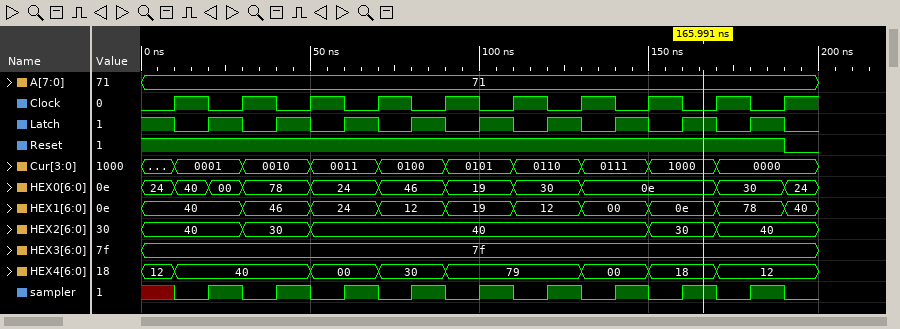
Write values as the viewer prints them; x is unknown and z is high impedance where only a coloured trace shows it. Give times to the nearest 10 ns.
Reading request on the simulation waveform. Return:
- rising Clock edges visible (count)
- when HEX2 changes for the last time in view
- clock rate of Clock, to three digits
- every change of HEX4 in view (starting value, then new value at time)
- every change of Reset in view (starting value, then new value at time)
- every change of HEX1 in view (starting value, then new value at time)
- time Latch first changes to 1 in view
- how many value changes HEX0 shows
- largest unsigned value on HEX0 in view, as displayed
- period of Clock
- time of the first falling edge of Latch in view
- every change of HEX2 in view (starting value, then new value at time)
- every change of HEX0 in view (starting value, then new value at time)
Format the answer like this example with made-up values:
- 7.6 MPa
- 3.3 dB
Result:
- 10
- 170 ns
- 50.0 MHz
- 12, 40 at 10 ns, 00 at 50 ns, 30 at 70 ns, 79 at 90 ns, 00 at 130 ns, 18 at 150 ns, 12 at 170 ns
- 1, 0 at 190 ns
- 40, 46 at 30 ns, 24 at 50 ns, 12 at 70 ns, 19 at 90 ns, 12 at 110 ns, 00 at 130 ns, 0e at 150 ns, 78 at 170 ns, 40 at 190 ns
- 20 ns
- 10
- 78
- 20 ns
- 10 ns
- 40, 30 at 30 ns, 40 at 50 ns, 30 at 150 ns, 40 at 170 ns
- 24, 40 at 10 ns, 00 at 20 ns, 78 at 30 ns, 24 at 50 ns, 46 at 70 ns, 19 at 90 ns, 30 at 110 ns, 0e at 130 ns, 30 at 170 ns, 24 at 190 ns
